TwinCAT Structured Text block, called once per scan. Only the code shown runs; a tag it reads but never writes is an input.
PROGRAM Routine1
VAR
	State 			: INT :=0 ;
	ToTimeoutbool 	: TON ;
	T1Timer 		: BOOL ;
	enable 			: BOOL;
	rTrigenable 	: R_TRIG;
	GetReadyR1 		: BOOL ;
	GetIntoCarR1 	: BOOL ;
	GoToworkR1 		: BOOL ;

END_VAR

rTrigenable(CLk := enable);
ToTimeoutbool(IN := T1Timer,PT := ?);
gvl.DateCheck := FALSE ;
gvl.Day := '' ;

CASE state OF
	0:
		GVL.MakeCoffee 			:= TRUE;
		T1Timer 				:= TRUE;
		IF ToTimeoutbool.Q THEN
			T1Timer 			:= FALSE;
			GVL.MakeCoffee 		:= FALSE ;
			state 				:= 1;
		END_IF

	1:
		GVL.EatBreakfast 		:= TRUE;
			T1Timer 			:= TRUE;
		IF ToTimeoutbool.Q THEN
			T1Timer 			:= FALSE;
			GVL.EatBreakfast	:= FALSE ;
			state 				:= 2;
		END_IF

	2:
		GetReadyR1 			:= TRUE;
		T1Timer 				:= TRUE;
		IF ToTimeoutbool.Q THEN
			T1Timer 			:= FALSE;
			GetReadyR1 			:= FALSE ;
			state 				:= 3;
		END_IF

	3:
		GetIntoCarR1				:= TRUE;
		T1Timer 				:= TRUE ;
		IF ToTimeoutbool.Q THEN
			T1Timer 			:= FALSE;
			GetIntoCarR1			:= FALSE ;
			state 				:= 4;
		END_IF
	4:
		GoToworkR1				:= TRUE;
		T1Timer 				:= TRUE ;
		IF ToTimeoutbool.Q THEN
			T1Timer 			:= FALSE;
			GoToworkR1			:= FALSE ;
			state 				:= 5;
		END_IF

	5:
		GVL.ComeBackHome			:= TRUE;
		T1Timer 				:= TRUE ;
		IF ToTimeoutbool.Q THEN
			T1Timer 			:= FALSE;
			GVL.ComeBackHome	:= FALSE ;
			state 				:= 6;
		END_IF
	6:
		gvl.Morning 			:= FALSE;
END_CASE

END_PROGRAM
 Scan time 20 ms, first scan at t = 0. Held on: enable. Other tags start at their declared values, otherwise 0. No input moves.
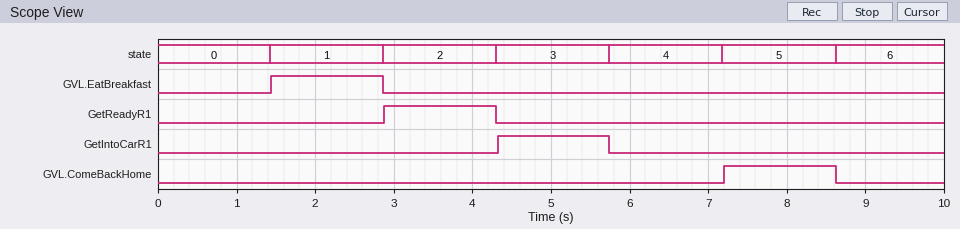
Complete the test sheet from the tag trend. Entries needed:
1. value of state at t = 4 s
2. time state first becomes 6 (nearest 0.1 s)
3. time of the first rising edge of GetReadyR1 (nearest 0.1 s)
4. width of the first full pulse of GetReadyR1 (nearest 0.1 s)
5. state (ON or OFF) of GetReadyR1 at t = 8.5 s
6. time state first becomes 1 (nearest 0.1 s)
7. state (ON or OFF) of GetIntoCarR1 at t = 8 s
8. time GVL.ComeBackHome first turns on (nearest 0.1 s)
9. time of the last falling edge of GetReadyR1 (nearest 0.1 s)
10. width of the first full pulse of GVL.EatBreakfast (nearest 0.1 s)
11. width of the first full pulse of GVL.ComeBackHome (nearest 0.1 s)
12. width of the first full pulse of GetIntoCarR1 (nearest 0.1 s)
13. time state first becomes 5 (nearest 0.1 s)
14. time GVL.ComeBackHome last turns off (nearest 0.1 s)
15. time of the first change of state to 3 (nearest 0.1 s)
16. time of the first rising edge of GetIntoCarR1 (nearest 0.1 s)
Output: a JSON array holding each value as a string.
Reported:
["2", "8.6 s", "2.9 s", "1.4 s", "OFF", "1.4 s", "OFF", "7.2 s", "4.3 s", "1.4 s", "1.4 s", "1.4 s", "7.2 s", "8.6 s", "4.3 s", "4.3 s"]
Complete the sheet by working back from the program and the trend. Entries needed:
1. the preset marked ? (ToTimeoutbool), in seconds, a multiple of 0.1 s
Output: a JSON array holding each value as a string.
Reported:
["1.4 s"]
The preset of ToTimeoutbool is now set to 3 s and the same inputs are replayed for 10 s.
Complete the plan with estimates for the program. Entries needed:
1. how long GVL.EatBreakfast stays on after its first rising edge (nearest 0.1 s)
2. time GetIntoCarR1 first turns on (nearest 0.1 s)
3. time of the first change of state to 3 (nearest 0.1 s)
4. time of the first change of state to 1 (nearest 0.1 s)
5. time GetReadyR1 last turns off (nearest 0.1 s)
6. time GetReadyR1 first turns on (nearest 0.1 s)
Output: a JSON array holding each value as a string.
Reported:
["3.0 s", "9.1 s", "9.1 s", "3.0 s", "9.1 s", "6.1 s"]
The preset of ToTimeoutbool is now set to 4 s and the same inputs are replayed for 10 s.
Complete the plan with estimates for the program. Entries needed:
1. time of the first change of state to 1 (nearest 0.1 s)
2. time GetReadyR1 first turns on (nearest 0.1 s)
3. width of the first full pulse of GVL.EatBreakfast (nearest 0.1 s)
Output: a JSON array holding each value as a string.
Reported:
["4.0 s", "8.1 s", "4.0 s"]
